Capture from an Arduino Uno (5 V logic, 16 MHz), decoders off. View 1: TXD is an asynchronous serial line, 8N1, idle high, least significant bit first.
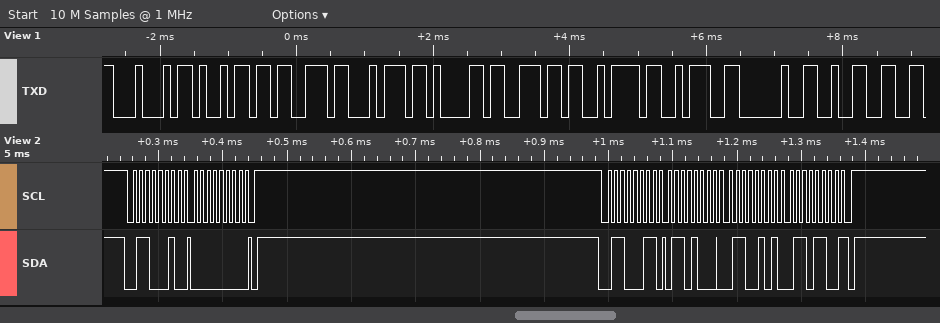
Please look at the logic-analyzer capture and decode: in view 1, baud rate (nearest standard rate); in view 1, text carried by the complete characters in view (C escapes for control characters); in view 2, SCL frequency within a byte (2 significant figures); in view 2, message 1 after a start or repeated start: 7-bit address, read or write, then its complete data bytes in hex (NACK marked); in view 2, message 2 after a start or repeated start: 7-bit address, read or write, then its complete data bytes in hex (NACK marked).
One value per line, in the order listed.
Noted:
9600 baud
"Distanz: 2"
100 kHz
0x31 write: 00
0x31 read: 68 65 6C NACK
